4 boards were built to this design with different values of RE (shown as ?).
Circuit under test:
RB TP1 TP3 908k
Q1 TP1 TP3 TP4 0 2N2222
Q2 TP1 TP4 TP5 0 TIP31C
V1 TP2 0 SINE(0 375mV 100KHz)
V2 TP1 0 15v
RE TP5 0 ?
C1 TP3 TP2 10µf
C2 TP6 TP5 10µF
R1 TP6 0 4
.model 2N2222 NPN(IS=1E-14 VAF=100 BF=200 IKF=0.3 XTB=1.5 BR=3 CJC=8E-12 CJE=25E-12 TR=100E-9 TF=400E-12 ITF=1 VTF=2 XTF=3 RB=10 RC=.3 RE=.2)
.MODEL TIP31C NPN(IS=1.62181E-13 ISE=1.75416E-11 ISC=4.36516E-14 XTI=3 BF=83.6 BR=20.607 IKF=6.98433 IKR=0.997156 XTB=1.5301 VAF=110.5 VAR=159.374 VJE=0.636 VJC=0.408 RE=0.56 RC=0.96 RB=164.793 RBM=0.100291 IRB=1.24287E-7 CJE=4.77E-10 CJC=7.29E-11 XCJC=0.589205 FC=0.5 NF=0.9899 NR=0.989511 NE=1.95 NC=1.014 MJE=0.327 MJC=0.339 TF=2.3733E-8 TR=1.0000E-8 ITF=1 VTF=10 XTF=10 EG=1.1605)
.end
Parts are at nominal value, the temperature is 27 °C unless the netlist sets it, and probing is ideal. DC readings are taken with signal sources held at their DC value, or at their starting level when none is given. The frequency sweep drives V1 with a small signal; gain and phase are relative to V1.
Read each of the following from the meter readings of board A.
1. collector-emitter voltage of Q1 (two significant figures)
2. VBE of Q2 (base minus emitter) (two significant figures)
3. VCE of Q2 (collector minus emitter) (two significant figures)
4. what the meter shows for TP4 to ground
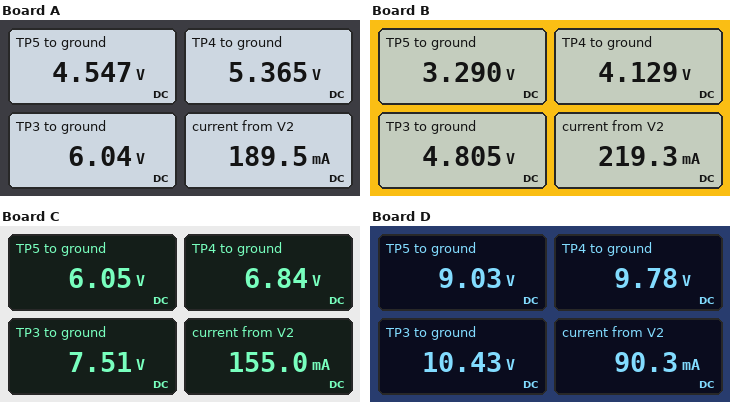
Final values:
9.6 V
820 mV
10 V
5.365 V
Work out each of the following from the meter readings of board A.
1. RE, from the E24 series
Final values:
24 Ω
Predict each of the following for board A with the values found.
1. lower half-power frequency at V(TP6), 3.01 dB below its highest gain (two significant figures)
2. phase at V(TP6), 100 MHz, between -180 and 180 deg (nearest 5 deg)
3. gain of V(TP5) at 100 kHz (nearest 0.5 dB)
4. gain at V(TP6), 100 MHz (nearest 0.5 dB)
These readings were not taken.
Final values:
3.3 kHz
-5 deg
-2.0 dB
-14.0 dB
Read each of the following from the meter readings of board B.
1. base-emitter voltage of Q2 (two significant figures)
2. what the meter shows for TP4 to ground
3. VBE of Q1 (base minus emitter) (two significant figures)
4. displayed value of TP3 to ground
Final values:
840 mV
4.129 V
680 mV
4.805 V
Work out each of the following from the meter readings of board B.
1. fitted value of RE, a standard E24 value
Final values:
15 Ω
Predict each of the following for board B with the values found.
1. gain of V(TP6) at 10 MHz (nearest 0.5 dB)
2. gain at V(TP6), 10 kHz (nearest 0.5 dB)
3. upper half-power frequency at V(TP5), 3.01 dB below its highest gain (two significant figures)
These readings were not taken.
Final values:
-13.0 dB
-2.5 dB
840 kHz
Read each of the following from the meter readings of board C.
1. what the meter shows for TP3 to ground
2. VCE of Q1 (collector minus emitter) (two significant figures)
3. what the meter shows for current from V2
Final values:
7.51 V
8.2 V
155.0 mA
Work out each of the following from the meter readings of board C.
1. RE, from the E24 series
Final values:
39 Ω
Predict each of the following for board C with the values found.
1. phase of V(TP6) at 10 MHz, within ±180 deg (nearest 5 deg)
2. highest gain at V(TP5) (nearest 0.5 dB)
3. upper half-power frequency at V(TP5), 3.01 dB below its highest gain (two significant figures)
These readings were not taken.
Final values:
-20 deg
0 dB
720 kHz
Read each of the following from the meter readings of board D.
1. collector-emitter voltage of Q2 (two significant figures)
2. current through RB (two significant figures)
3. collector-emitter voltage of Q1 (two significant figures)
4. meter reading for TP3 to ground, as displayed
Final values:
6.0 V
5.0 µA
5.2 V
10.43 V
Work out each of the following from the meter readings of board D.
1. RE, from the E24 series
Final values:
100 Ω
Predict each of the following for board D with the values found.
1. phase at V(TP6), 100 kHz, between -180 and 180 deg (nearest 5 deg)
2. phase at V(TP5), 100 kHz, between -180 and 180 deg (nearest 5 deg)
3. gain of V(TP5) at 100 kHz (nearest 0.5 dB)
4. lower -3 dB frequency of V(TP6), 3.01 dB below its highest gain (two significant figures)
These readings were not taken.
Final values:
-5 deg
-5 deg
-2.5 dB
3.1 kHz
